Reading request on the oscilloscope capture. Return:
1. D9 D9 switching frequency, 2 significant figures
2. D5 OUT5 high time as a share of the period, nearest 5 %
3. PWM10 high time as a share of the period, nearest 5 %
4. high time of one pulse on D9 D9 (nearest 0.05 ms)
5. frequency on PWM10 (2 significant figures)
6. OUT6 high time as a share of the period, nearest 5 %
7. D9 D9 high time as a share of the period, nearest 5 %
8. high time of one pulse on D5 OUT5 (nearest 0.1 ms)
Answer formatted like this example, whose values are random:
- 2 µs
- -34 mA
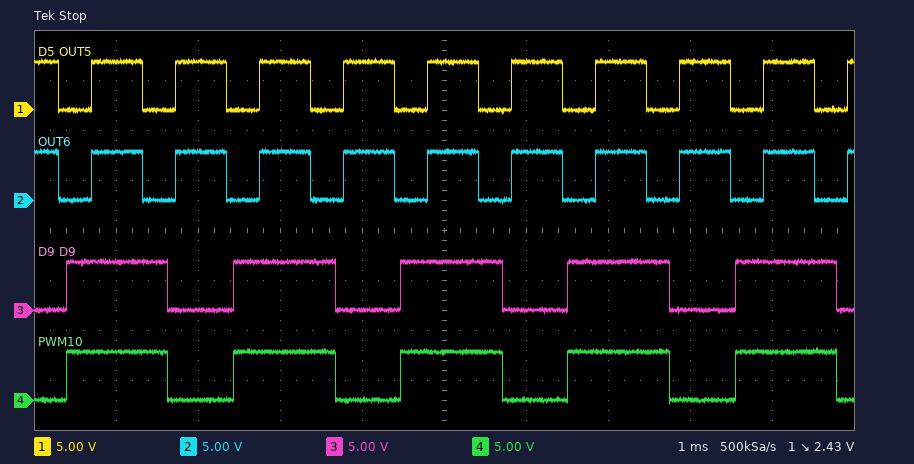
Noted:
- 490 Hz
- 60 %
- 60 %
- 1.25 ms
- 490 Hz
- 60 %
- 60 %
- 0.6 ms
